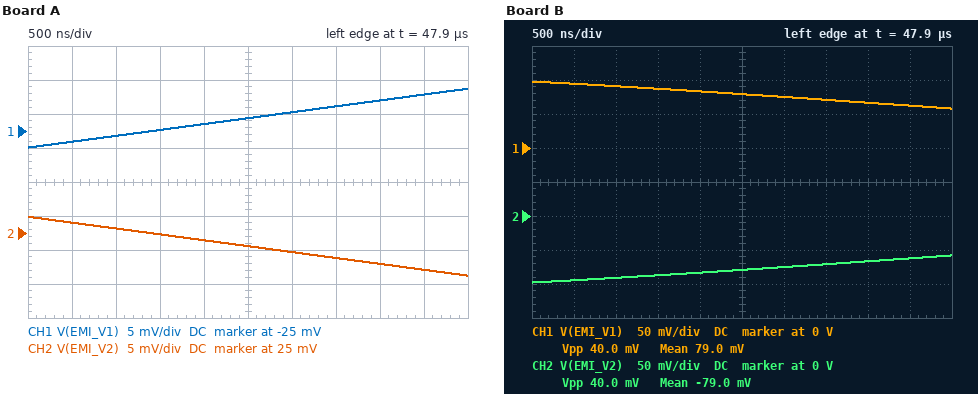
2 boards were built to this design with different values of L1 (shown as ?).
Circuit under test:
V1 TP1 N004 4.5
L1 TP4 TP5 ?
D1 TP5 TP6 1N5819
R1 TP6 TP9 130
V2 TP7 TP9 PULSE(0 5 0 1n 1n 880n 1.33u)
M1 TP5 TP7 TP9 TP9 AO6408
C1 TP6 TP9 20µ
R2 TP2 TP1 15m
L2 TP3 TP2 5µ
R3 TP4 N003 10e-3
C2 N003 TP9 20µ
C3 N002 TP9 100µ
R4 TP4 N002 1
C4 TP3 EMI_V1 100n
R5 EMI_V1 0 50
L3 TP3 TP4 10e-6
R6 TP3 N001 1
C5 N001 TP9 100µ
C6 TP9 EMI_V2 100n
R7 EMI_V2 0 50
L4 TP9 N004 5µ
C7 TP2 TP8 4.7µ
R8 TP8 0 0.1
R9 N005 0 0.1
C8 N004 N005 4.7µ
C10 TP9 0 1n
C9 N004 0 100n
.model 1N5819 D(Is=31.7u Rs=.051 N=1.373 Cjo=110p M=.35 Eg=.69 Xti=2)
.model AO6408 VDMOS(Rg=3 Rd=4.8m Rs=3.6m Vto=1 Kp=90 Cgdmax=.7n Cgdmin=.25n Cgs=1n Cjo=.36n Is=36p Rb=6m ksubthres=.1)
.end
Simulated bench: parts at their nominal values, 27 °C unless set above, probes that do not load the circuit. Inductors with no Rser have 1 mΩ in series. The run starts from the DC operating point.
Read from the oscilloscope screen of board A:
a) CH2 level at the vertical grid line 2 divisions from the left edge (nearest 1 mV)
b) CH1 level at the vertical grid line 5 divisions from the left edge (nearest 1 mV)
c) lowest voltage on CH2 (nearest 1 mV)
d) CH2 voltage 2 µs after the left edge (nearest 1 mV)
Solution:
26 mV
-23 mV
19 mV
24 mV
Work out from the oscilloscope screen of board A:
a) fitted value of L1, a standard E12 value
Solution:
33 µH
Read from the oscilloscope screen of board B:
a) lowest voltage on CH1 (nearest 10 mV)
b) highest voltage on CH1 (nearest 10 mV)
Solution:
60 mV
100 mV
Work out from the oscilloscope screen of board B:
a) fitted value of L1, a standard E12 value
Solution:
3.3 µH
